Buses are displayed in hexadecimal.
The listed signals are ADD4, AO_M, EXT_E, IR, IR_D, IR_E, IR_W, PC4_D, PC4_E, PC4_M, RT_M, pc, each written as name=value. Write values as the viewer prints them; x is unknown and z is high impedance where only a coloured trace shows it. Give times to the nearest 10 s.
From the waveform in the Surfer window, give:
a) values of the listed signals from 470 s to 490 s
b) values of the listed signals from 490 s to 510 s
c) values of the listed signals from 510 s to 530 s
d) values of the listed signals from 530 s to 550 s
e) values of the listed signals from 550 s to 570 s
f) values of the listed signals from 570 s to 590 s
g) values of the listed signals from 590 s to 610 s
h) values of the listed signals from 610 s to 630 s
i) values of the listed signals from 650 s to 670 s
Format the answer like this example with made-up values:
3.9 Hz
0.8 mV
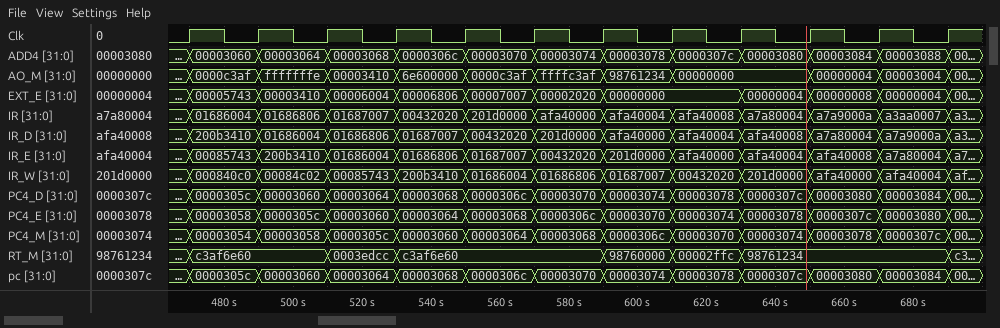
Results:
ADD4=00003060, AO_M=0000c3af, EXT_E=00005743, IR=01686004, IR_D=200b3410, IR_E=00085743, IR_W=000840c0, PC4_D=0000305c, PC4_E=00003058, PC4_M=00003054, RT_M=c3af6e60, pc=0000305c
ADD4=00003064, AO_M=fffffffe, EXT_E=00003410, IR=01686806, IR_D=01686004, IR_E=200b3410, IR_W=00084c02, PC4_D=00003060, PC4_E=0000305c, PC4_M=00003058, RT_M=c3af6e60, pc=00003060
ADD4=00003068, AO_M=00003410, EXT_E=00006004, IR=01687007, IR_D=01686806, IR_E=01686004, IR_W=00085743, PC4_D=00003064, PC4_E=00003060, PC4_M=0000305c, RT_M=0003edcc, pc=00003064
ADD4=0000306c, AO_M=6e600000, EXT_E=00006806, IR=00432020, IR_D=01687007, IR_E=01686806, IR_W=200b3410, PC4_D=00003068, PC4_E=00003064, PC4_M=00003060, RT_M=c3af6e60, pc=00003068
ADD4=00003070, AO_M=0000c3af, EXT_E=00007007, IR=201d0000, IR_D=00432020, IR_E=01687007, IR_W=01686004, PC4_D=0000306c, PC4_E=00003068, PC4_M=00003064, RT_M=c3af6e60, pc=0000306c
ADD4=00003074, AO_M=ffffc3af, EXT_E=00002020, IR=afa40000, IR_D=201d0000, IR_E=00432020, IR_W=01686806, PC4_D=00003070, PC4_E=0000306c, PC4_M=00003068, RT_M=c3af6e60, pc=00003070
ADD4=00003078, AO_M=98761234, EXT_E=00000000, IR=afa40004, IR_D=afa40000, IR_E=201d0000, IR_W=01687007, PC4_D=00003074, PC4_E=00003070, PC4_M=0000306c, RT_M=98760000, pc=00003074
ADD4=0000307c, AO_M=00000000, EXT_E=00000000, IR=afa40008, IR_D=afa40004, IR_E=afa40000, IR_W=00432020, PC4_D=00003078, PC4_E=00003074, PC4_M=00003070, RT_M=00002ffc, pc=00003078
ADD4=00003084, AO_M=00000004, EXT_E=00000008, IR=a7a9000a, IR_D=a7a80004, IR_E=afa40008, IR_W=afa40000, PC4_D=00003080, PC4_E=0000307c, PC4_M=00003078, RT_M=98761234, pc=00003080
